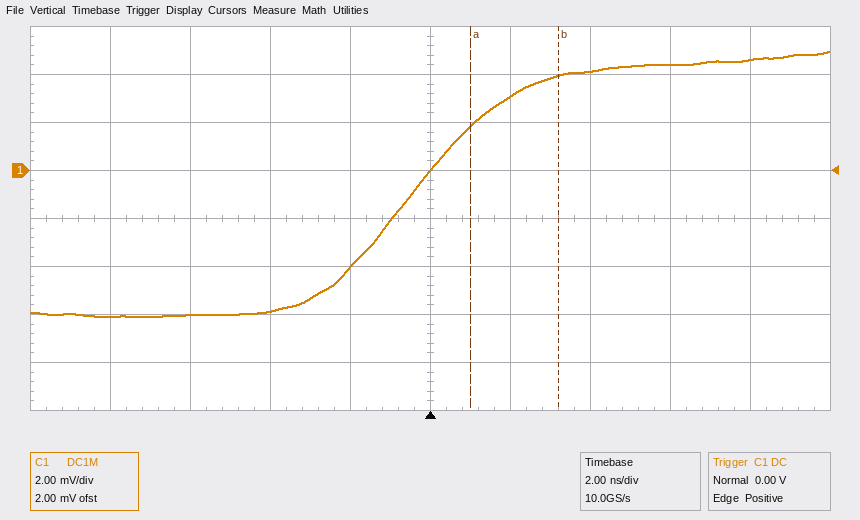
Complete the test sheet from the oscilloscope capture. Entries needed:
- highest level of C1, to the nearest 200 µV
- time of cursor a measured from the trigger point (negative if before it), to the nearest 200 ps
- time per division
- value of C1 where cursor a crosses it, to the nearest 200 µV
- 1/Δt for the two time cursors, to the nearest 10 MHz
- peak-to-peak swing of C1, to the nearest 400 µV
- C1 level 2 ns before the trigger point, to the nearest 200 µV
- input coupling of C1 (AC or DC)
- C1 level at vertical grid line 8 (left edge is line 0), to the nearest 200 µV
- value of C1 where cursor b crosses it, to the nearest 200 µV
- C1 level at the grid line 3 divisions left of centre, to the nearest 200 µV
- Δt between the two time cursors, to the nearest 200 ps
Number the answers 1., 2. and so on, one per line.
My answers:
1. 5.0 mV
2. +1.0 ns
3. 2 ns
4. 1.8 mV
5. 450 MHz
6. 11.2 mV
7. -4.0 mV
8. DC
9. 4.4 mV
10. 4.0 mV
11. -6.0 mV
12. 2.2 ns
